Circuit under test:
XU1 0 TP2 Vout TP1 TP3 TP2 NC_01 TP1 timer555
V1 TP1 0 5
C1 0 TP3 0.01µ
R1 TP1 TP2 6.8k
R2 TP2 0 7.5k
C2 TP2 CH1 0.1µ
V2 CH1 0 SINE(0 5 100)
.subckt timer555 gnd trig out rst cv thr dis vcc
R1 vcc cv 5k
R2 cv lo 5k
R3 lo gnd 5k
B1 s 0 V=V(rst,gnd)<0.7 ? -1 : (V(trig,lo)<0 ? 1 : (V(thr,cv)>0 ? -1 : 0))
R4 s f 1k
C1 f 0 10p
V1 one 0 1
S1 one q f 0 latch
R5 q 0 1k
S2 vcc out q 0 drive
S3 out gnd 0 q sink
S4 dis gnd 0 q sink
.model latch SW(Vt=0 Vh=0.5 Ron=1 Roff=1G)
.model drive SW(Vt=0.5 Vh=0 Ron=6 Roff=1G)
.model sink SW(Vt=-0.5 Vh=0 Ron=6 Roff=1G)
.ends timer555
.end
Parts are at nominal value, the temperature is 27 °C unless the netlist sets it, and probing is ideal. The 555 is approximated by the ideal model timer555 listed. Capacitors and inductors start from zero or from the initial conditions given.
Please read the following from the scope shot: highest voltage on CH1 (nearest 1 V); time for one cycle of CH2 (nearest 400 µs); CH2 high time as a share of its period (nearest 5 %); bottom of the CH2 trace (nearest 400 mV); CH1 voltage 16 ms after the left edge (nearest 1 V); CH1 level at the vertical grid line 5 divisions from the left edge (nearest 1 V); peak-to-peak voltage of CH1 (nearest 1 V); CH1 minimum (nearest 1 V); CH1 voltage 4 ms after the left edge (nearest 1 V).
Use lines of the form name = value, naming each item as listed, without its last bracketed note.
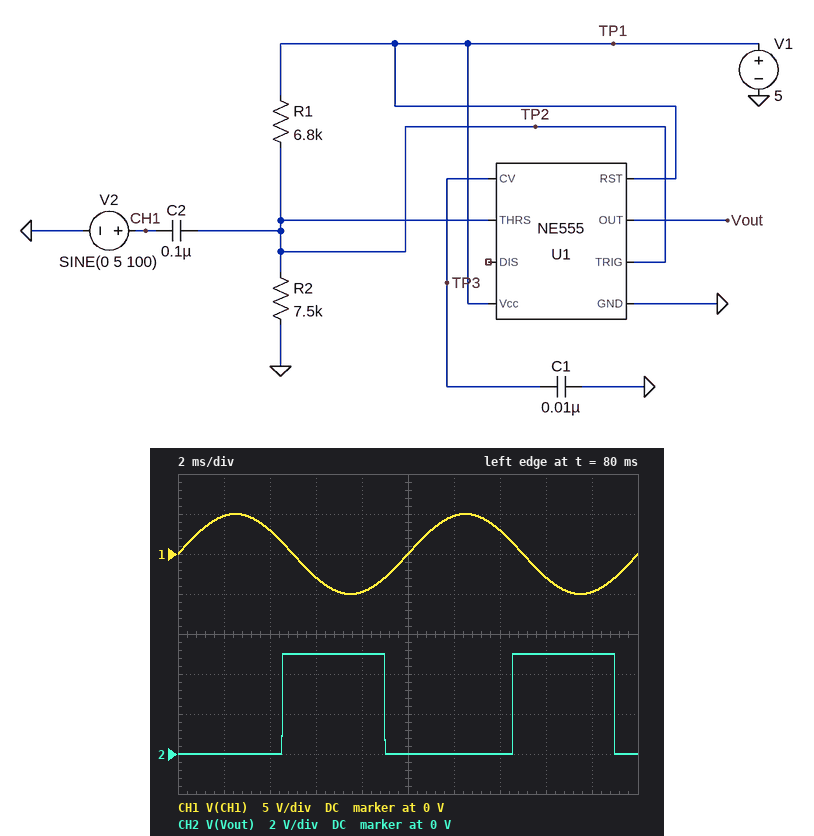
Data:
highest voltage on CH1 = 5 V
time for one cycle of CH2 = 10.0 ms
CH2 high time as a share of its period = 45 %
bottom of the CH2 trace = 0 V
CH1 voltage 16 ms after the left edge = -3 V
CH1 level at the vertical grid line 5 divisions from the left edge = 0 V
peak-to-peak voltage of CH1 = 10 V
CH1 minimum = -5 V
CH1 voltage 4 ms after the left edge = 3 V
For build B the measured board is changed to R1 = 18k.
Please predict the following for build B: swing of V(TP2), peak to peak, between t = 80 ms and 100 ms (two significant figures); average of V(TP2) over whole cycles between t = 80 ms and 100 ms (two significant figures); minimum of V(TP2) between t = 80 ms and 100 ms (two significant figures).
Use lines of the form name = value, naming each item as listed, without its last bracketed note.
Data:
swing of V(TP2), peak to peak, between t = 80 ms and 100 ms = 3.2 V
average of V(TP2) over whole cycles between t = 80 ms and 100 ms = 1.5 V
minimum of V(TP2) between t = 80 ms and 100 ms = -110 mV
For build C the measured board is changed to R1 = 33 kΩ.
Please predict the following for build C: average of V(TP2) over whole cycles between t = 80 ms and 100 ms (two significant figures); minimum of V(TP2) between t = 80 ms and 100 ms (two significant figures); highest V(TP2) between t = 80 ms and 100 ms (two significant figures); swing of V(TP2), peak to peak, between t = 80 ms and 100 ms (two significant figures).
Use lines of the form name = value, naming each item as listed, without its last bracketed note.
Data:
average of V(TP2) over whole cycles between t = 80 ms and 100 ms = 930 mV
minimum of V(TP2) between t = 80 ms and 100 ms = -870 mV
highest V(TP2) between t = 80 ms and 100 ms = 2.7 V
swing of V(TP2), peak to peak, between t = 80 ms and 100 ms = 3.6 V
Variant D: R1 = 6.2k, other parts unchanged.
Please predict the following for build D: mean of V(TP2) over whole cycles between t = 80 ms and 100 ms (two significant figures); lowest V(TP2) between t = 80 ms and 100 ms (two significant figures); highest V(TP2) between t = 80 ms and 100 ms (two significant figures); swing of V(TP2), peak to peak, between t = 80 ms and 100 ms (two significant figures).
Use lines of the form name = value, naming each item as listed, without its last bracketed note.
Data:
mean of V(TP2) over whole cycles between t = 80 ms and 100 ms = 2.7 V
lowest V(TP2) between t = 80 ms and 100 ms = 1.7 V
highest V(TP2) between t = 80 ms and 100 ms = 3.8 V
swing of V(TP2), peak to peak, between t = 80 ms and 100 ms = 2.1 V
